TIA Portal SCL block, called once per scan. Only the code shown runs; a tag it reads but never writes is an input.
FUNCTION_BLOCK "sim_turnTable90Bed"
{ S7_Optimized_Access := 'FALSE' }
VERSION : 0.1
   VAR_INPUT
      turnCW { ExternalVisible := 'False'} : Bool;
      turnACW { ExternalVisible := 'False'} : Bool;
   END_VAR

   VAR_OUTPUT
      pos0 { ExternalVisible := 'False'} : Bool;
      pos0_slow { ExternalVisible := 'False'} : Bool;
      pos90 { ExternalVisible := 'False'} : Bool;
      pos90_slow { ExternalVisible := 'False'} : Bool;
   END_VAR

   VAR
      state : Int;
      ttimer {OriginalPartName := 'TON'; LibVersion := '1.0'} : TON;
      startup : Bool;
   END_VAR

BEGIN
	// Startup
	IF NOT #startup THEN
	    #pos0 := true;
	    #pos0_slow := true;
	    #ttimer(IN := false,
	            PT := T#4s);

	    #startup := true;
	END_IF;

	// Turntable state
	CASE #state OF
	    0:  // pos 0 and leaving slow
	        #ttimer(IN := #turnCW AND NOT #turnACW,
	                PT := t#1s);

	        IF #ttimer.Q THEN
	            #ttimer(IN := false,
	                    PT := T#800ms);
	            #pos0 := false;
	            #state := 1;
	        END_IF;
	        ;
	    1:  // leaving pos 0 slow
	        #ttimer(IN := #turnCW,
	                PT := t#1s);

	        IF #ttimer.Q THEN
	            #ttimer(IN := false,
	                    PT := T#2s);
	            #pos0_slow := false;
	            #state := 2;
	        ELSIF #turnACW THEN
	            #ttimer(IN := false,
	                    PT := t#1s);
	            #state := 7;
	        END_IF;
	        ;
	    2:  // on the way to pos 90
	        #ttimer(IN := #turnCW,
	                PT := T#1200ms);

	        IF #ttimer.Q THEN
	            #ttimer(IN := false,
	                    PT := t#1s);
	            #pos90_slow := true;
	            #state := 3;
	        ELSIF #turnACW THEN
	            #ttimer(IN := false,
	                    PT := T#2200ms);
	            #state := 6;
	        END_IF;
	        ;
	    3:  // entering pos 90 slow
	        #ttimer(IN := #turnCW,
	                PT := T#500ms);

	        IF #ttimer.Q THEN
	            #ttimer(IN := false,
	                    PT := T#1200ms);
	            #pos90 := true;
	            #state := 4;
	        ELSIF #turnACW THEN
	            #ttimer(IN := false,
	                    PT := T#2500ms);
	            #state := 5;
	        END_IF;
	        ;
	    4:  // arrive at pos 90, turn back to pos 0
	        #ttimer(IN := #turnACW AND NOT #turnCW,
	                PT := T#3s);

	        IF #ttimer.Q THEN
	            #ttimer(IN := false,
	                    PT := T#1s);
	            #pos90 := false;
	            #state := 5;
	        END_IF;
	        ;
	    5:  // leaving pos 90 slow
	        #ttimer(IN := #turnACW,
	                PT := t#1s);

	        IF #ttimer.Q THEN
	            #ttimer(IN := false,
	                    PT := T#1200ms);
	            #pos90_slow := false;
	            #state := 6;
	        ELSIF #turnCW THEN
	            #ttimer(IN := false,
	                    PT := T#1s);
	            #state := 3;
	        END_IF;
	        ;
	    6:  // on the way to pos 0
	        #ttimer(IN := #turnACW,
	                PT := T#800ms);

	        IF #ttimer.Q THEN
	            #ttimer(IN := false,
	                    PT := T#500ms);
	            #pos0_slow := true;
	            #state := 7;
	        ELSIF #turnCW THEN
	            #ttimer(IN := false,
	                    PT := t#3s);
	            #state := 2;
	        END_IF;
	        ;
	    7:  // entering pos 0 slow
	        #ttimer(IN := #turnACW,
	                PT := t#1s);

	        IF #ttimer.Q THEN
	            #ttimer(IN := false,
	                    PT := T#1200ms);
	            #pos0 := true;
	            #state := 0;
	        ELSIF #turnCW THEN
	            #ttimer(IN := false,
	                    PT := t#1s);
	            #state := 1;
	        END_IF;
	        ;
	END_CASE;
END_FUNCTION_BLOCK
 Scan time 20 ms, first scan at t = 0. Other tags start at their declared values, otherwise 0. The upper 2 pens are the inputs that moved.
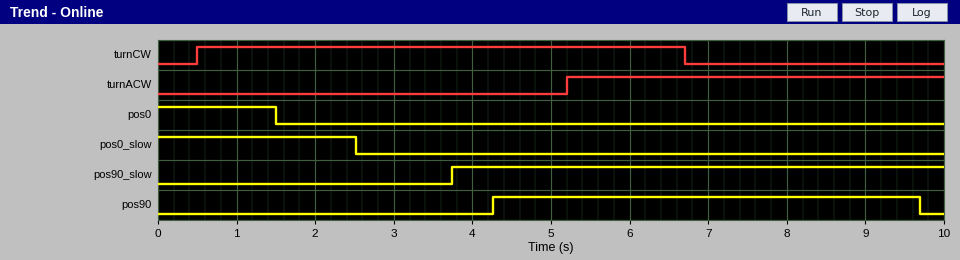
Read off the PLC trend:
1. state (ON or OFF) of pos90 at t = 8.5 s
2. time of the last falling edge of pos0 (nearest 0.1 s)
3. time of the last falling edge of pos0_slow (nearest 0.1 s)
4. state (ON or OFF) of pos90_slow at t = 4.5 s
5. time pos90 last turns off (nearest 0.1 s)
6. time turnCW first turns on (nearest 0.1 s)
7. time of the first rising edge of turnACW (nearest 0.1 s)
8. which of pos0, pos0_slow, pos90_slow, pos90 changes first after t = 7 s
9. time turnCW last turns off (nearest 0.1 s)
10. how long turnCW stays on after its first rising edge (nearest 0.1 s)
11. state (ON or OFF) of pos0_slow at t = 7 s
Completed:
ON
1.5 s
2.5 s
ON
9.7 s
0.5 s
5.2 s
pos90
6.7 s
6.2 s
OFF
